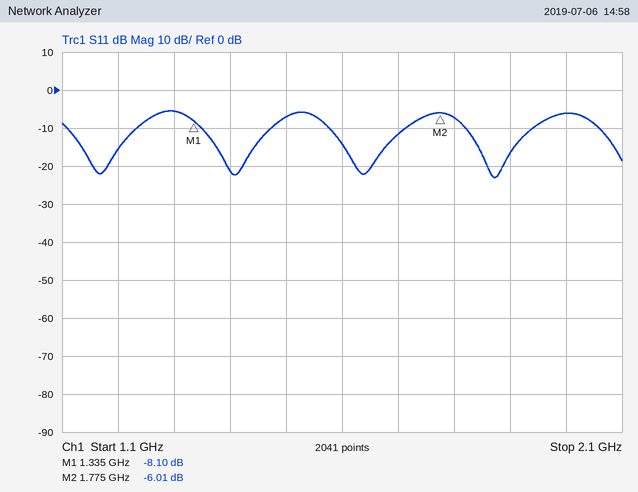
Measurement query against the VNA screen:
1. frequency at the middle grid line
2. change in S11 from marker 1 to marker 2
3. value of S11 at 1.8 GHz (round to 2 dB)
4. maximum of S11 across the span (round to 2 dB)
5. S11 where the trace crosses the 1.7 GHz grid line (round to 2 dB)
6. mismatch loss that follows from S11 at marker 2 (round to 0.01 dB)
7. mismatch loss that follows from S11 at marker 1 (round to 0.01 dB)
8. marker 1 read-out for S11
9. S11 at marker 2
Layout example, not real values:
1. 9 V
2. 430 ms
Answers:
1. 1.6 GHz
2. 2.09 dB
3. -8 dB
4. -6 dB
5. -12 dB
6. 1.25 dB
7. 0.73 dB
8. -8.10 dB
9. -6.01 dB
